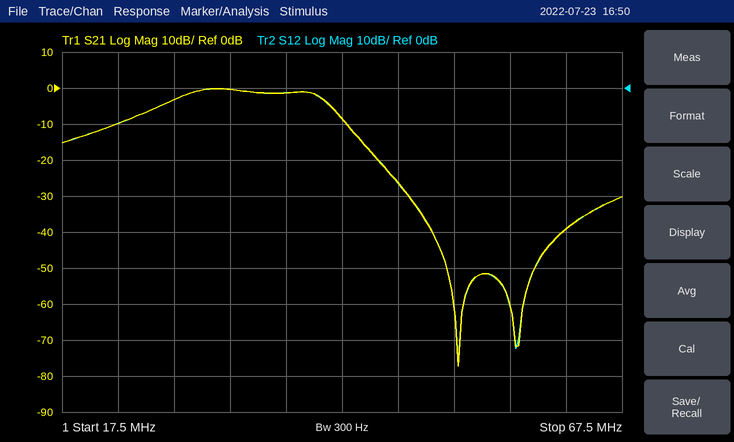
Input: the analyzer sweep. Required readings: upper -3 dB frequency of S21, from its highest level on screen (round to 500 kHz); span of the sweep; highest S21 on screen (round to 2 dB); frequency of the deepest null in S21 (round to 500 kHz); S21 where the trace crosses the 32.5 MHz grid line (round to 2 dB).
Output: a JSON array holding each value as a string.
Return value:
["41.0 MHz", "50 MHz", "0 dB", "53.0 MHz", "0 dB"]
